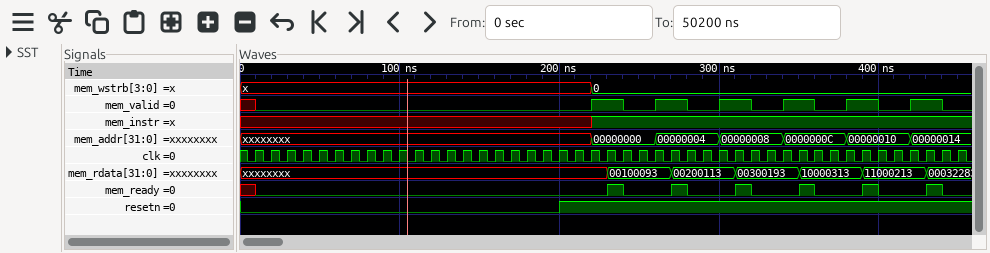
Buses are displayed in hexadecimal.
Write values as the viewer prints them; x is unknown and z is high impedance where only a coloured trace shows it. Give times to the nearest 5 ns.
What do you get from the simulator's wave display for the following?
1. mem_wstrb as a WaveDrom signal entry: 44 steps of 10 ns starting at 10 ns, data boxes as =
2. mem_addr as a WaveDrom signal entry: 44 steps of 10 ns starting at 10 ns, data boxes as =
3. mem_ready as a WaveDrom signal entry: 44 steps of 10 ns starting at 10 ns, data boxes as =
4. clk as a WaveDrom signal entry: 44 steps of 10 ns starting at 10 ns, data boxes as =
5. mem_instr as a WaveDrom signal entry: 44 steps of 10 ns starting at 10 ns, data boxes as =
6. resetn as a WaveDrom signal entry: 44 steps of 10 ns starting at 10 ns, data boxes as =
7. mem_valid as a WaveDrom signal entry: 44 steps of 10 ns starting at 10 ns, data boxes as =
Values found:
{name: 'mem_wstrb', wave: 'x....................=......................', data: '0'}
{name: 'mem_addr', wave: 'x....................=...=...=...=...=...=..', data: '00000000 00000004 00000008 0000000C 00000010 00000014'}
{name: 'mem_ready', wave: '0.....................10..10..10..10..10..10'}
{name: 'clk', wave: 'p...........................................'}
{name: 'mem_instr', wave: 'x....................1......................'}
{name: 'resetn', wave: '0..................1........................'}
{name: 'mem_valid', wave: '0....................1.0.1.0.1.0.1.0.1.0.1.0'}
